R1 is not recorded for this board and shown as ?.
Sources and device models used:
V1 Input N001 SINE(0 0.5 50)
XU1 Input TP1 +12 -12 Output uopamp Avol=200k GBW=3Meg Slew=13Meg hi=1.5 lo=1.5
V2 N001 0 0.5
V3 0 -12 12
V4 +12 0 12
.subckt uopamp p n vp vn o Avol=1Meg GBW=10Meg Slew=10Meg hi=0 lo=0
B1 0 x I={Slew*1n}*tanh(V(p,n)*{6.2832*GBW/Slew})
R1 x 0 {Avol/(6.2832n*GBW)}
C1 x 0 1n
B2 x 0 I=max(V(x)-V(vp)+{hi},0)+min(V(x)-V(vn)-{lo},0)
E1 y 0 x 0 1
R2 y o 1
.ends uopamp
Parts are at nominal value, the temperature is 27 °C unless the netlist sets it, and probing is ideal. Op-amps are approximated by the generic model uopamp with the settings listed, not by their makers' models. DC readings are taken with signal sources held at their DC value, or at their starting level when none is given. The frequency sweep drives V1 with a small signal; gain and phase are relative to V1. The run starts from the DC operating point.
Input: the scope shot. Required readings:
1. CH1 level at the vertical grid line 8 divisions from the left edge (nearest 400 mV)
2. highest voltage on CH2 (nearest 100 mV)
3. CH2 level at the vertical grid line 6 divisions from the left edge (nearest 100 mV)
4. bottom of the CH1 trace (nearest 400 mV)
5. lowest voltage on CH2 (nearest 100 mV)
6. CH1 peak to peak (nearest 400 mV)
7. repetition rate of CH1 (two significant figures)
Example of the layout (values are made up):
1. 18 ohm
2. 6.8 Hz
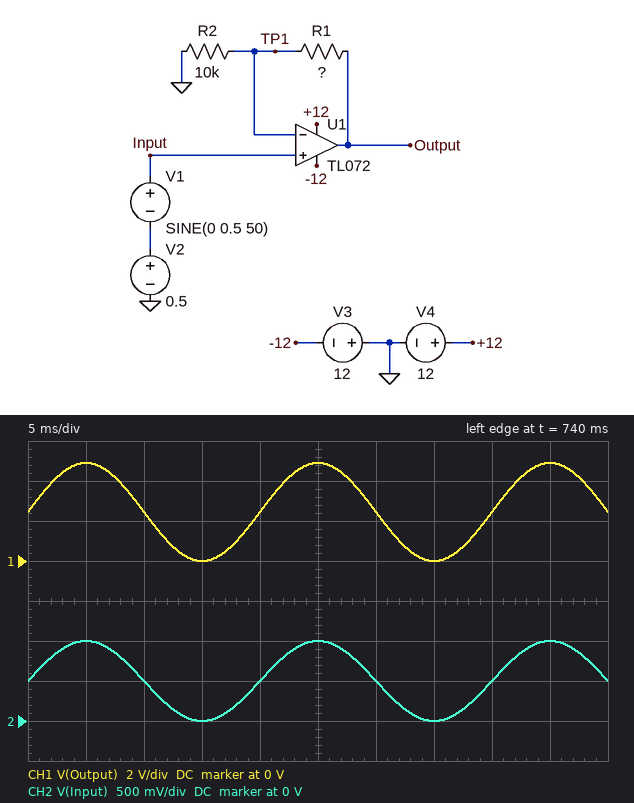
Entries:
1. 2.4 V
2. 1.0 V
3. 500 mV
4. 0 V
5. 0 V
6. 4.8 V
7. 50 Hz
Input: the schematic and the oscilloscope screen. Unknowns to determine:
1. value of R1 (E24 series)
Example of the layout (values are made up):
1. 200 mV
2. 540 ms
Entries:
1. 39 kΩ
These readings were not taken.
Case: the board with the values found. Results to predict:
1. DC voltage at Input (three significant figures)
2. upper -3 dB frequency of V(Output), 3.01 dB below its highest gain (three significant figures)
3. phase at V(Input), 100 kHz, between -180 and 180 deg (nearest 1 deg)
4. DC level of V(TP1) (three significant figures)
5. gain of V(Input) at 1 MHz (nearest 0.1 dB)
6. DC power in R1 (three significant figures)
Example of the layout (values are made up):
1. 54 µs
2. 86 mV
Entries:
1. 500 mV
2. 612 kHz
3. 0 deg
4. 500 mV
5. 0 dB
6. 97.5 µW
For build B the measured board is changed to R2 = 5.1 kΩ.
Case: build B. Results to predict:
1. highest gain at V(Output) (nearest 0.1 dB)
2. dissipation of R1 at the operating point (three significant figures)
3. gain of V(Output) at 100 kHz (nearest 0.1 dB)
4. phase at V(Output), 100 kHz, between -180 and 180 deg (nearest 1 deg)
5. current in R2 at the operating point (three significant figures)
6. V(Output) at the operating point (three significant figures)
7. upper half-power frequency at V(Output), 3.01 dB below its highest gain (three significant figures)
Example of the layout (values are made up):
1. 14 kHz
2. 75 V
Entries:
1. 18.7 dB
2. 375 µW
3. 18.4 dB
4. -16 deg
5. 98.0 µA
6. 4.32 V
7. 347 kHz
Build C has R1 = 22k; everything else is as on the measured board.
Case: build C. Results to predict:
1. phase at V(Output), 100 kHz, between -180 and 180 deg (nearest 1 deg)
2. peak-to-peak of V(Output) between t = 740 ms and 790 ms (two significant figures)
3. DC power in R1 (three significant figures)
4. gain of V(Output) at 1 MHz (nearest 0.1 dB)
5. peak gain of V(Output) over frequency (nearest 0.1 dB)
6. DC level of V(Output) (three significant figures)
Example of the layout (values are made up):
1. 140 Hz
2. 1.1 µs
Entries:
1. -6 deg
2. 3.2 V
3. 55.0 µW
4. 6.8 dB
5. 10.1 dB
6. 1.60 V
